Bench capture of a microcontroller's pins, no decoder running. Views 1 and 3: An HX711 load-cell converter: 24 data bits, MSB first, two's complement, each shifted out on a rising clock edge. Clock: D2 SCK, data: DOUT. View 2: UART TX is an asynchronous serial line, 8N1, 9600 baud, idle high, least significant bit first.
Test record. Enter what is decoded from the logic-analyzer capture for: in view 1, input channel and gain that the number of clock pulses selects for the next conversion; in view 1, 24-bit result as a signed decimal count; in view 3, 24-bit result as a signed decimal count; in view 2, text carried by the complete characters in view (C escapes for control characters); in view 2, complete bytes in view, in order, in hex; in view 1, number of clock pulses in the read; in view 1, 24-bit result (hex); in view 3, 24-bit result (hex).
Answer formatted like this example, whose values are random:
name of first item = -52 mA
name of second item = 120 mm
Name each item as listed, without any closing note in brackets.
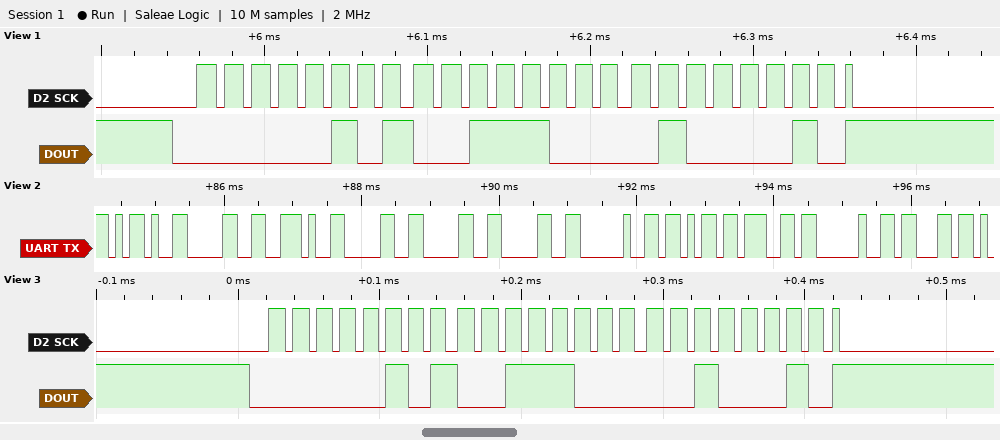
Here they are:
in view 1, input channel and gain that the number of clock pulses selects for the next conversion = channel A, gain 128
in view 1, 24-bit result as a signed decimal count = 342082
in view 3, 24-bit result as a signed decimal count = 342050
in view 2, text carried by the complete characters in view = "-0.000 kg c"
in view 2, complete bytes in view, in order, in hex = 2D 30 2E 30 30 30 20 6B 67 20 63
in view 1, number of clock pulses in the read = 25
in view 1, 24-bit result = 0x053842
in view 3, 24-bit result = 0x053822
